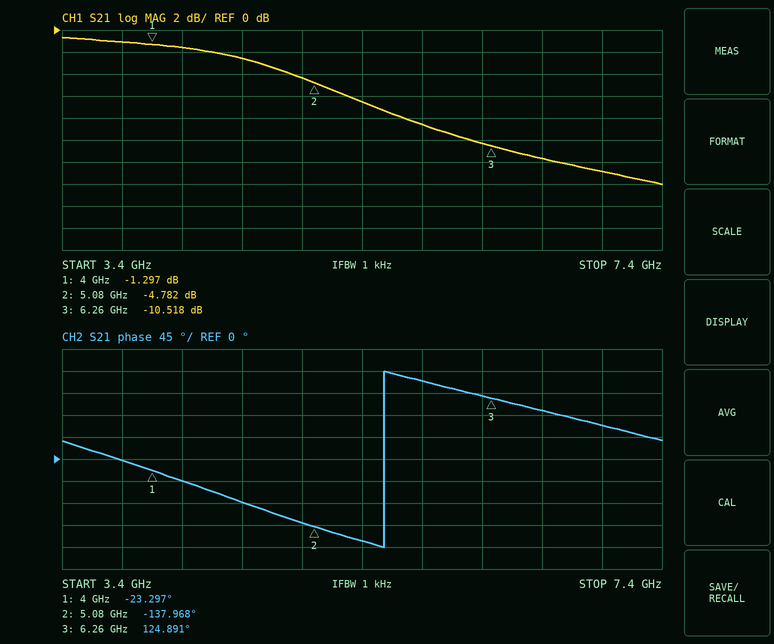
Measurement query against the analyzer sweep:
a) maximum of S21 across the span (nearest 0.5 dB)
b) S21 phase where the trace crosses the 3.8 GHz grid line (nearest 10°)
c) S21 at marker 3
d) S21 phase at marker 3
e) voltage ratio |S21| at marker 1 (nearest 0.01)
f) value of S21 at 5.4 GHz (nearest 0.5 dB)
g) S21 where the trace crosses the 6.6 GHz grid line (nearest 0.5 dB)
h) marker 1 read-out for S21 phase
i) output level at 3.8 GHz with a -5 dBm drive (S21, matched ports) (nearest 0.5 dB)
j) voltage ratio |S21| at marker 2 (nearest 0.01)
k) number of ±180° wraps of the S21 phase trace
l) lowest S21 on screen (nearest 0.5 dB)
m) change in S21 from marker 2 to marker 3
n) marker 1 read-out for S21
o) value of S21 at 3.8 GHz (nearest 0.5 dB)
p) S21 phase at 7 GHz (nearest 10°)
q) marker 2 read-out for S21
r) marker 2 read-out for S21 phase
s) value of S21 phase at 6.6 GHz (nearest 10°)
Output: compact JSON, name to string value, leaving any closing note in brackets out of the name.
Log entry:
{"maximum of S21 across the span": "-0.5 dB", "S21 phase where the trace crosses the 3.8 GHz grid line": "0°", "S21 at marker 3": "-10.518 dB", "S21 phase at marker 3": "124.891°", "voltage ratio |S21| at marker 1": "0.86", "value of S21 at 5.4 GHz": "-6.5 dB", "S21 where the trace crosses the 6.6 GHz grid line": "-11.5 dB", "marker 1 read-out for S21 phase": "-23.297°", "output level at 3.8 GHz with a -5 dBm drive (S21, matched ports)": "-6.0 dBm", "voltage ratio |S21| at marker 2": "0.58", "number of ±180° wraps of the S21 phase trace": "1", "lowest S21 on screen": "-14.0 dB", "change in S21 from marker 2 to marker 3": "-5.736 dB", "marker 1 read-out for S21": "-1.297 dB", "value of S21 at 3.8 GHz": "-1.0 dB", "S21 phase at 7 GHz": "70°", "marker 2 read-out for S21": "-4.782 dB", "marker 2 read-out for S21 phase": "-137.968°", "value of S21 phase at 6.6 GHz": "100°"}
